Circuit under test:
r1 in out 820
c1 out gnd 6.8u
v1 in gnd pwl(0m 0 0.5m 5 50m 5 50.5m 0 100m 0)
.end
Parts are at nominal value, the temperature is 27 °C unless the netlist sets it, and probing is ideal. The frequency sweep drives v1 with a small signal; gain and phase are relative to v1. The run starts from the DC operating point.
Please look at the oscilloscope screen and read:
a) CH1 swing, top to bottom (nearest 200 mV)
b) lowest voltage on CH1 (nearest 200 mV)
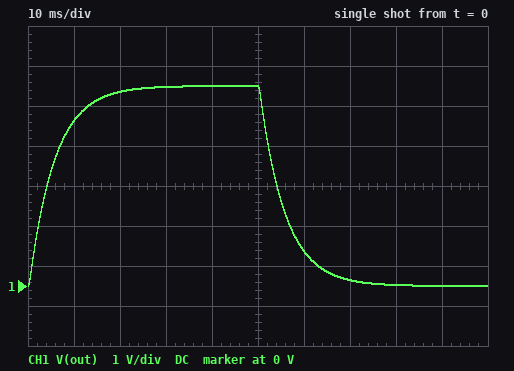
5.0 V
0 V
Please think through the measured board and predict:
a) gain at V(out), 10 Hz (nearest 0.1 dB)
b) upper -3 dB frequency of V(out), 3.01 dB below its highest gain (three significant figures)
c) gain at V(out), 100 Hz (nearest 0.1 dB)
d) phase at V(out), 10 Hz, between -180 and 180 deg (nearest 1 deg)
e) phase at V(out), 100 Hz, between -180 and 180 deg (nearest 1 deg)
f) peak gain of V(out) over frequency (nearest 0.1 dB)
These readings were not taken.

-0.5 dB
28.5 Hz
-11.2 dB
-19 deg
-74 deg
0 dB
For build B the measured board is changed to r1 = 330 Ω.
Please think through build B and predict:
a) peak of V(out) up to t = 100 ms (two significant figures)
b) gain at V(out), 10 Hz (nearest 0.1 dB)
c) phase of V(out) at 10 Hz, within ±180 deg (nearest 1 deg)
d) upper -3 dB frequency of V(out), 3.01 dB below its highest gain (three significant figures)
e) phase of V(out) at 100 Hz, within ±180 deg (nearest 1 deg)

5.0 V
-0.1 dB
-8 deg
70.9 Hz
-55 deg
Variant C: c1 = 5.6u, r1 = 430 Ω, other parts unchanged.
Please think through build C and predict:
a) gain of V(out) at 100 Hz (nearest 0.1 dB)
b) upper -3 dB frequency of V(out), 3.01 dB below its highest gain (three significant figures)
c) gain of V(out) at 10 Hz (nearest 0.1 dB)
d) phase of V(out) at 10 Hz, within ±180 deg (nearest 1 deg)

-5.2 dB
66.1 Hz
-0.1 dB
-9 deg
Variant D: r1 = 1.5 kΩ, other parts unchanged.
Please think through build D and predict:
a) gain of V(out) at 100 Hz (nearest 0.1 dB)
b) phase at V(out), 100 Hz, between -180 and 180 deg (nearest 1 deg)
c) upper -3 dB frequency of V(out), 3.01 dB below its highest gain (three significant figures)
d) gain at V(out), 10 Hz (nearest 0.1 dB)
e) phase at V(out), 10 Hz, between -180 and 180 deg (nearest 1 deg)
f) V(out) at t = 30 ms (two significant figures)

-16.2 dB
-81 deg
15.6 Hz
-1.5 dB
-33 deg
4.7 V
